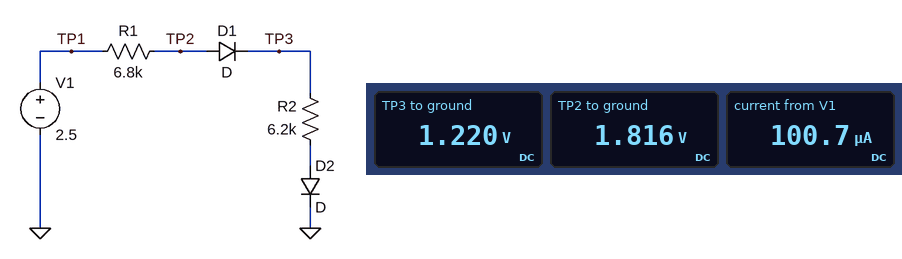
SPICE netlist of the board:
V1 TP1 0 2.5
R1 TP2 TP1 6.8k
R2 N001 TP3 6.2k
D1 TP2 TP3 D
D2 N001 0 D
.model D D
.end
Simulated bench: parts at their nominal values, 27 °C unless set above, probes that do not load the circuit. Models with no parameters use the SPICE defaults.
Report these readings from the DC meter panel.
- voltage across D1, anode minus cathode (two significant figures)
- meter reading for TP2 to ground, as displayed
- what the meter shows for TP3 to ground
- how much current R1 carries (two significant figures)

600 mV
1.816 V
1.220 V
100 µA
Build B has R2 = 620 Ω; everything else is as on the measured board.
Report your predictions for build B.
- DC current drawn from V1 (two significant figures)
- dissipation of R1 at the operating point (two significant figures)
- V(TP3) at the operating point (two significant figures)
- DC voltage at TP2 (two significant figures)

170 µA
200 µW
720 mV
1.3 V
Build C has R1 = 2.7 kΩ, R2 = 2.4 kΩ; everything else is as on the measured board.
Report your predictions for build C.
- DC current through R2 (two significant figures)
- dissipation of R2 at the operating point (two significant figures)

250 µA
150 µW
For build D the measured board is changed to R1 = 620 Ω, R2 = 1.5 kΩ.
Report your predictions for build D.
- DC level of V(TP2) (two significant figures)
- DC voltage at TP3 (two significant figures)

2.1 V
1.5 V
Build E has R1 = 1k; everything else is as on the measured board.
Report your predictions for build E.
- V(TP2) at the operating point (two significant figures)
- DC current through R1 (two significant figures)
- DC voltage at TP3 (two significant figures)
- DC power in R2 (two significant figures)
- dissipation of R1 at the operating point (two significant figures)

2.3 V
180 µA
1.7 V
200 µW
32 µW
